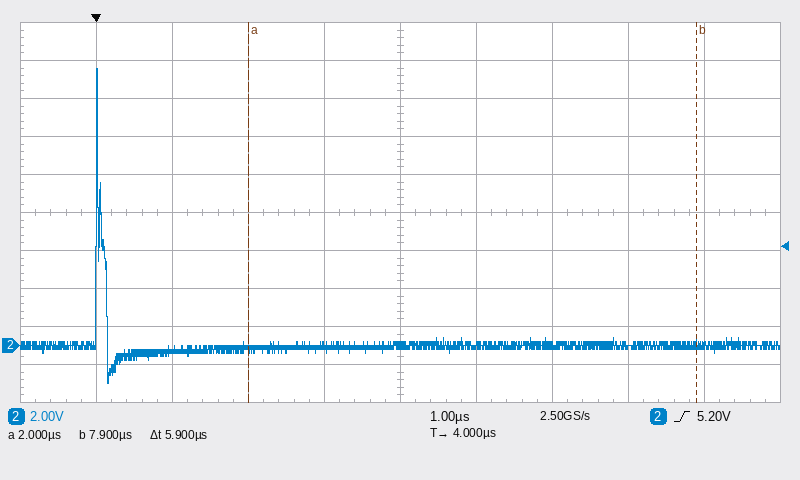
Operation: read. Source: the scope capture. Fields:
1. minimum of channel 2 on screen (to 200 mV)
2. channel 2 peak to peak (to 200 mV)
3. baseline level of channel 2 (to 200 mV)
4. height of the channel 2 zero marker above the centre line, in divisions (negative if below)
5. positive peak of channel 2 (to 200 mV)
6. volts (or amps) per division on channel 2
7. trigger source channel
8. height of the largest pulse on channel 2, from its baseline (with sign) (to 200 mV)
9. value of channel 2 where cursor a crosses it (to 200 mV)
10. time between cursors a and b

-2.0 V
16.6 V
0.0 V
-3.5 div
14.6 V
2 V
channel 2
+14.6 V
-200 mV
5.9 µs
